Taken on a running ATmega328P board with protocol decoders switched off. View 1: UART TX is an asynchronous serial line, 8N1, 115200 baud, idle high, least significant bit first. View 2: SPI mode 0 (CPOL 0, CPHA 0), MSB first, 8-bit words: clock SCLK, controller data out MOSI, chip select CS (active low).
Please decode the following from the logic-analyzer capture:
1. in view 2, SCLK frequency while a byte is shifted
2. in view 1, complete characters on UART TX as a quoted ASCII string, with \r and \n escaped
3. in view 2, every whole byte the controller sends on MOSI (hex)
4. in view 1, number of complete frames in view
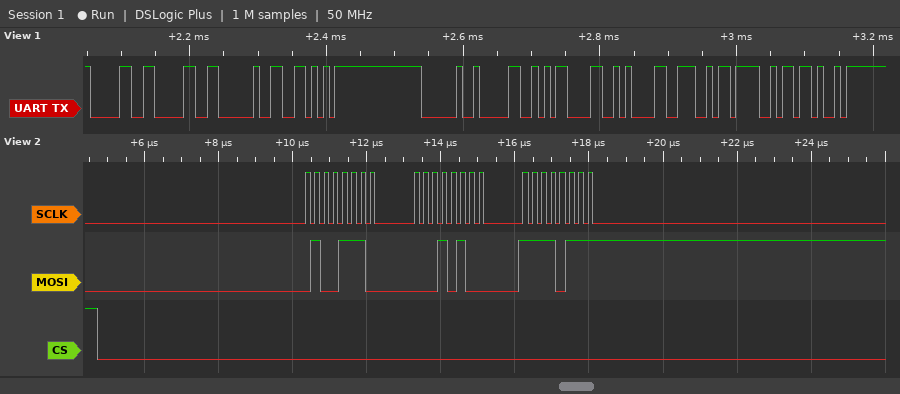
4 MHz
"00 V 0\r\nNOK"
4E 14 F7
11
